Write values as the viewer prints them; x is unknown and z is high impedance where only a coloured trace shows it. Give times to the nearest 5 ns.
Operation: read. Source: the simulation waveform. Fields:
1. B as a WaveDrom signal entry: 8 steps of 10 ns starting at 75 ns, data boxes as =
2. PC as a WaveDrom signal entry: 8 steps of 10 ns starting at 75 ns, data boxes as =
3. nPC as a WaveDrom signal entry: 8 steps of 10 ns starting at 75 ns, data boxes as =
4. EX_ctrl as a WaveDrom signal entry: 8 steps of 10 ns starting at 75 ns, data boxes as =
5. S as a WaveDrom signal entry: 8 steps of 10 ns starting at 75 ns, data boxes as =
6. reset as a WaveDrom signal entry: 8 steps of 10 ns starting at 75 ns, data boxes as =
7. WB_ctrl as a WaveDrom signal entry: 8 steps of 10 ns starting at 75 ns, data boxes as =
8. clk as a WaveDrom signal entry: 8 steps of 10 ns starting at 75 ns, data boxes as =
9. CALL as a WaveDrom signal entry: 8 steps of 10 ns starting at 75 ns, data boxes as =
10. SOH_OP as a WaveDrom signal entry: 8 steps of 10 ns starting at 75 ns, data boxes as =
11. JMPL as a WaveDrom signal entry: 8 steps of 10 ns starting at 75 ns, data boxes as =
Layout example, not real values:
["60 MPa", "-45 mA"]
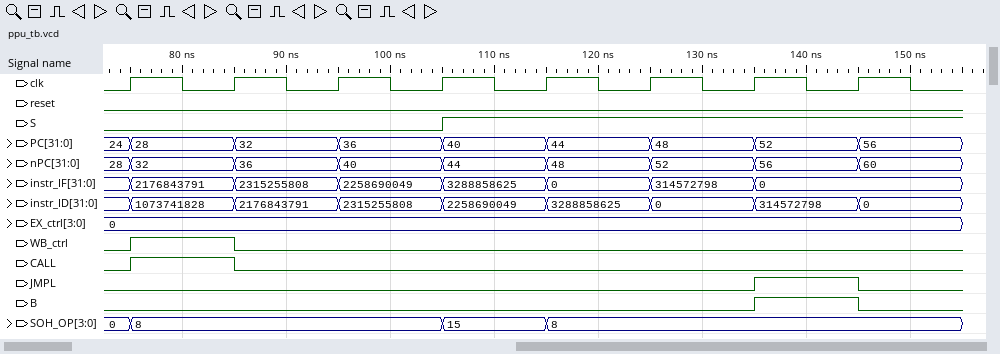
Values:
["{name: 'B', wave: '0.....10'}", "{name: 'PC', wave: '========', data: '28 32 36 40 44 48 52 56'}", "{name: 'nPC', wave: '========', data: '32 36 40 44 48 52 56 60'}", "{name: 'EX_ctrl', wave: '=.......', data: '0'}", "{name: 'S', wave: '0..1....'}", "{name: 'reset', wave: '0.......'}", "{name: 'WB_ctrl', wave: '10......'}", "{name: 'clk', wave: 'p.......'}", "{name: 'CALL', wave: '10......'}", "{name: 'SOH_OP', wave: '=..==...', data: '8 15 8'}", "{name: 'JMPL', wave: '0.....10'}"]
